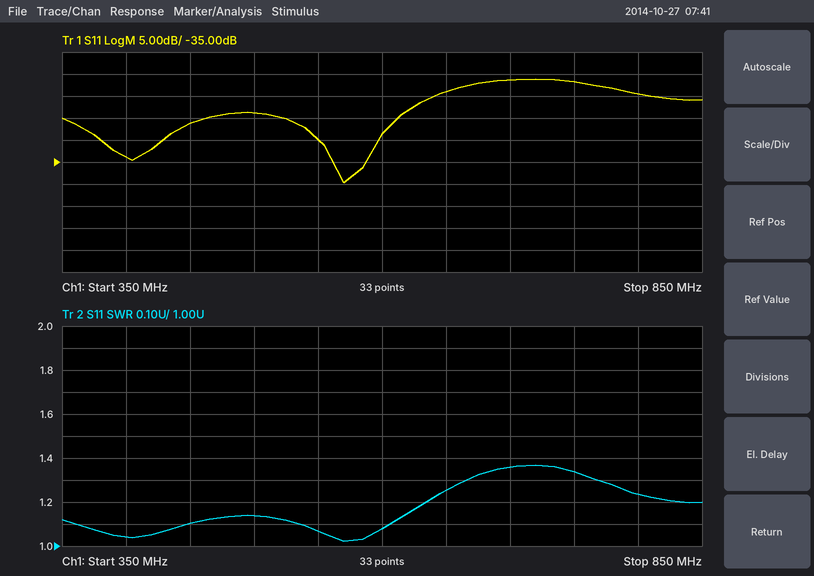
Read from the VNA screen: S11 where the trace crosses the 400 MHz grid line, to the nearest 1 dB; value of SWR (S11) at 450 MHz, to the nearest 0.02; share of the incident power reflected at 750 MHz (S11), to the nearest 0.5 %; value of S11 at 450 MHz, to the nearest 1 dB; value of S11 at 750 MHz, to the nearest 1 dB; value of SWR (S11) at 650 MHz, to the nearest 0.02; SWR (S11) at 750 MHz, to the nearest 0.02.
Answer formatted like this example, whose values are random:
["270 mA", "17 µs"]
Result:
["-34 dB", "1.10", "2.0 %", "-26 dB", "-17 dB", "1.26", "1.34"]
